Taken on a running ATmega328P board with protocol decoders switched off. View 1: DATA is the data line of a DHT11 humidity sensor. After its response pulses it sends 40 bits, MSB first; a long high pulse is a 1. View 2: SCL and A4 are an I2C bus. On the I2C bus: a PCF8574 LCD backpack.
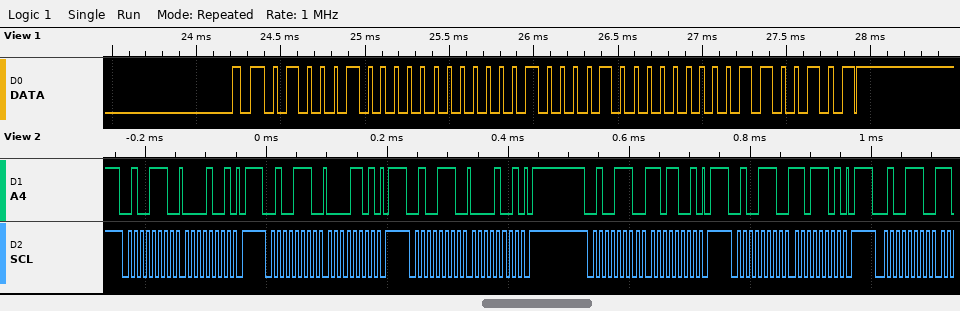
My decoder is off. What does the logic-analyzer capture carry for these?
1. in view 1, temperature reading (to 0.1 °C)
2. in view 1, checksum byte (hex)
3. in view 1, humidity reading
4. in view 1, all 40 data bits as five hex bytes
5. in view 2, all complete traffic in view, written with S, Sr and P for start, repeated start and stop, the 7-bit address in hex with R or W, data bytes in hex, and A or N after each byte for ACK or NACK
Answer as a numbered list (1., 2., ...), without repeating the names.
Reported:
1. 33.0 °C
2. 0x65
3. 68 %
4. 44 00 21 00 65
5. S 27W A 09 A P S 27W A 0D A P S 27W A 09 A P S 27W A D9 A P S 27W A DD A P S 27W A
